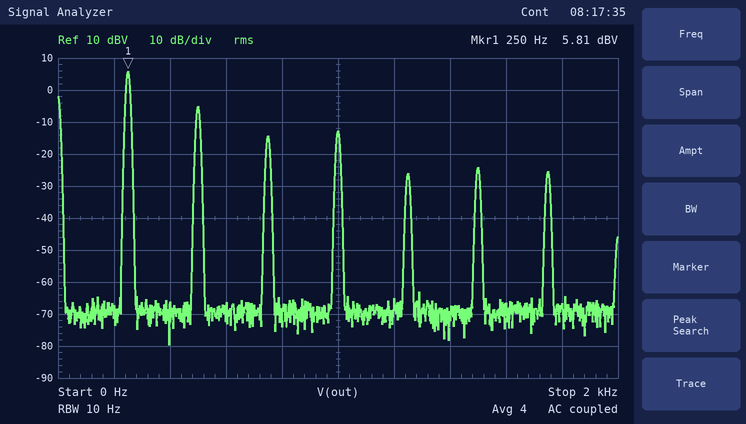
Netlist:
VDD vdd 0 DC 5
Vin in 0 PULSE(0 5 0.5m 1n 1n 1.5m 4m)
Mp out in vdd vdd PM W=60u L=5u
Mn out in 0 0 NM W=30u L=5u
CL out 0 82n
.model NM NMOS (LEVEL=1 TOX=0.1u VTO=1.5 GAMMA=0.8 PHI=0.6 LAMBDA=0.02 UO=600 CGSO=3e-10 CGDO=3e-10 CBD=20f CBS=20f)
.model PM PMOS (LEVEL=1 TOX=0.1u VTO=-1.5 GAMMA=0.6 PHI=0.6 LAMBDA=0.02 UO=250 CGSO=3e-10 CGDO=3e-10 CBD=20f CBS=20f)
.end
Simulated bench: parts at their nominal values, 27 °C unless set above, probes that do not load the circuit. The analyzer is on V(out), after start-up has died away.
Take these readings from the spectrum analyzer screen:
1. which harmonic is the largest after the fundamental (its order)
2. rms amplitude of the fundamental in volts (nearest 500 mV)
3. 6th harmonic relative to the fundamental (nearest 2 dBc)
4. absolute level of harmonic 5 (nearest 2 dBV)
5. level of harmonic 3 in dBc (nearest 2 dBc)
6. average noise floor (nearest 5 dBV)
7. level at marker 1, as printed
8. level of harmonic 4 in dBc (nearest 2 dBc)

2
2.0 V
-30 dBc
-26 dBV
-20 dBc
-70 dBV
5.81 dBV
-18 dBc
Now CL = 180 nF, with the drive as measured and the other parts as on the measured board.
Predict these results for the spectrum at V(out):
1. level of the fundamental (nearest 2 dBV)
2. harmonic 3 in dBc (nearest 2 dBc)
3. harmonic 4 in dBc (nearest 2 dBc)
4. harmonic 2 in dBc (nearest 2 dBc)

4 dBV
-28 dBc
-26 dBc
-14 dBc
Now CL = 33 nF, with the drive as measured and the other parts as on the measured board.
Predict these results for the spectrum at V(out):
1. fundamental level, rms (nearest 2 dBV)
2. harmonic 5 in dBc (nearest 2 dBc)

6 dBV
-26 dBc
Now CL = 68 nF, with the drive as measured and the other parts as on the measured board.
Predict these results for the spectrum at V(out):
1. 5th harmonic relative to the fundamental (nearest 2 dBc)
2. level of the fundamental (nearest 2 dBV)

-30 dBc
6 dBV
